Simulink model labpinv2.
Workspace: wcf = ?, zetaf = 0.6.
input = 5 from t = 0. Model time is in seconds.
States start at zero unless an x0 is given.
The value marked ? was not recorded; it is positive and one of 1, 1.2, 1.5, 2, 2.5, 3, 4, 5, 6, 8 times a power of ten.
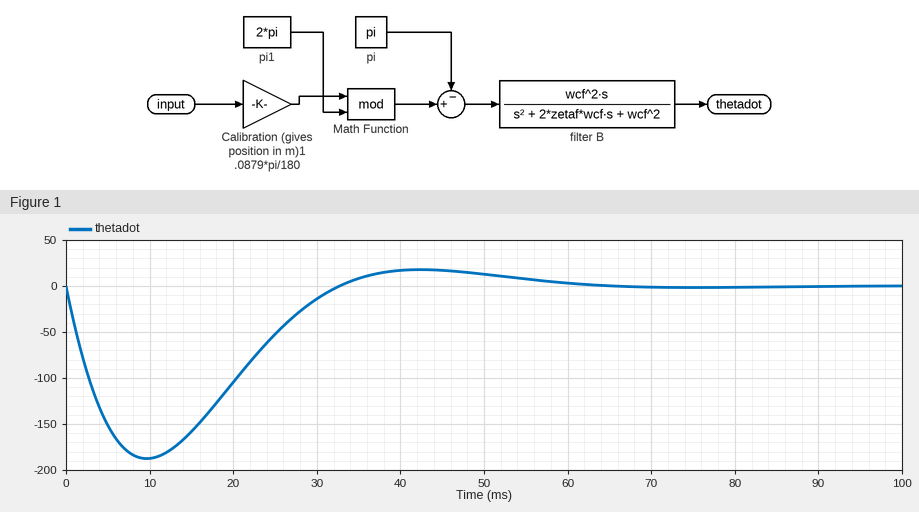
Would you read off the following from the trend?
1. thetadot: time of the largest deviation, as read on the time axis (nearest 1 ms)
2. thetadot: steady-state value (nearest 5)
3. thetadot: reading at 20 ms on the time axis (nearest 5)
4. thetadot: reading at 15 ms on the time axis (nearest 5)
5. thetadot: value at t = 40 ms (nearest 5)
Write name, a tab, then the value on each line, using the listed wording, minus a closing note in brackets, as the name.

thetadot: time of the largest deviation, as read on the time axis	10 ms
thetadot: steady-state value	0
thetadot: reading at 20 ms on the time axis	-105
thetadot: reading at 15 ms on the time axis	-160
thetadot: value at t = 40 ms	15
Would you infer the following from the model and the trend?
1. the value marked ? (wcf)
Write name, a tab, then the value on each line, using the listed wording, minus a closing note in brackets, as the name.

the value marked ?	120
